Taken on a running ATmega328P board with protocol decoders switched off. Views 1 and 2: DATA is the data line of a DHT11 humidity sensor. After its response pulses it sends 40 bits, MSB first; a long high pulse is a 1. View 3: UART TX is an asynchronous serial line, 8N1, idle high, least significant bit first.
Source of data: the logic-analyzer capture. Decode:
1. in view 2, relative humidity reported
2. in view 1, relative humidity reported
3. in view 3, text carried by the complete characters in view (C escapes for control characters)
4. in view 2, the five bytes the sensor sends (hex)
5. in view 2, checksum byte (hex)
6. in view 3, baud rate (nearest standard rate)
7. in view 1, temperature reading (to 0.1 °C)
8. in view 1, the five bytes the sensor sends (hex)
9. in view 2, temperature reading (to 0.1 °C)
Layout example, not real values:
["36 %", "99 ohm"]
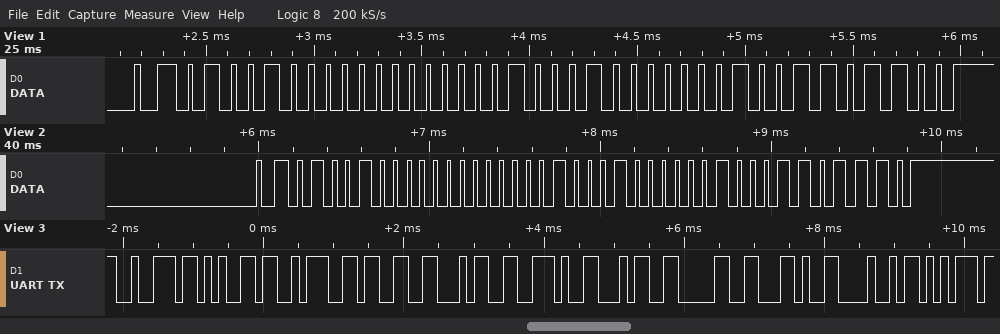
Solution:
["72 %", "72 %", "\"re:34.40,Hu\"", "48 00 22 04 6E", "0x6E", "9600 baud", "34.2 °C", "48 00 22 02 6C", "34.4 °C"]
